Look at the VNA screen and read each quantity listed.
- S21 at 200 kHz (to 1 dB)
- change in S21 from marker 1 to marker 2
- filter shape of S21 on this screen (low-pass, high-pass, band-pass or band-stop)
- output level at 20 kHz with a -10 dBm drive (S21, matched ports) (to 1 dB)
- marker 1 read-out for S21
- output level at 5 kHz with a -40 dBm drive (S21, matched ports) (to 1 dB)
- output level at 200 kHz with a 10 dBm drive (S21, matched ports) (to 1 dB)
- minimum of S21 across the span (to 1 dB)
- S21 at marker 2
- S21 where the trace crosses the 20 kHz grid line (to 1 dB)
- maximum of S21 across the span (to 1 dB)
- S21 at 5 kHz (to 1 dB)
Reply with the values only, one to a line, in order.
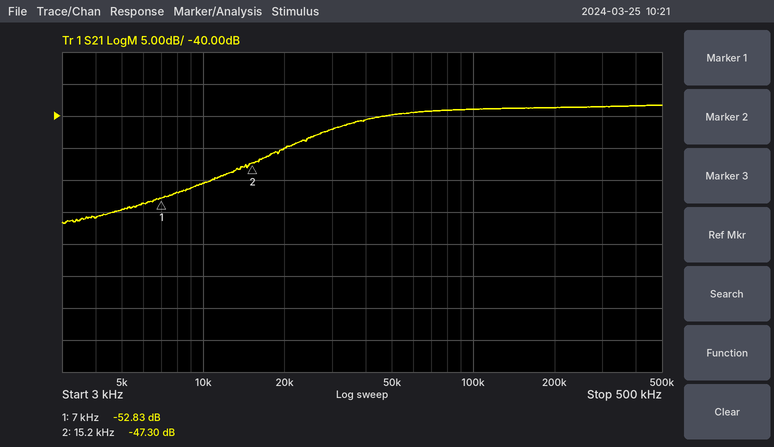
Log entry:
-39 dB
5.53 dB
high-pass
-55 dBm
-52.83 dB
-95 dBm
-29 dBm
-57 dB
-47.30 dB
-45 dB
-38 dB
-55 dB
